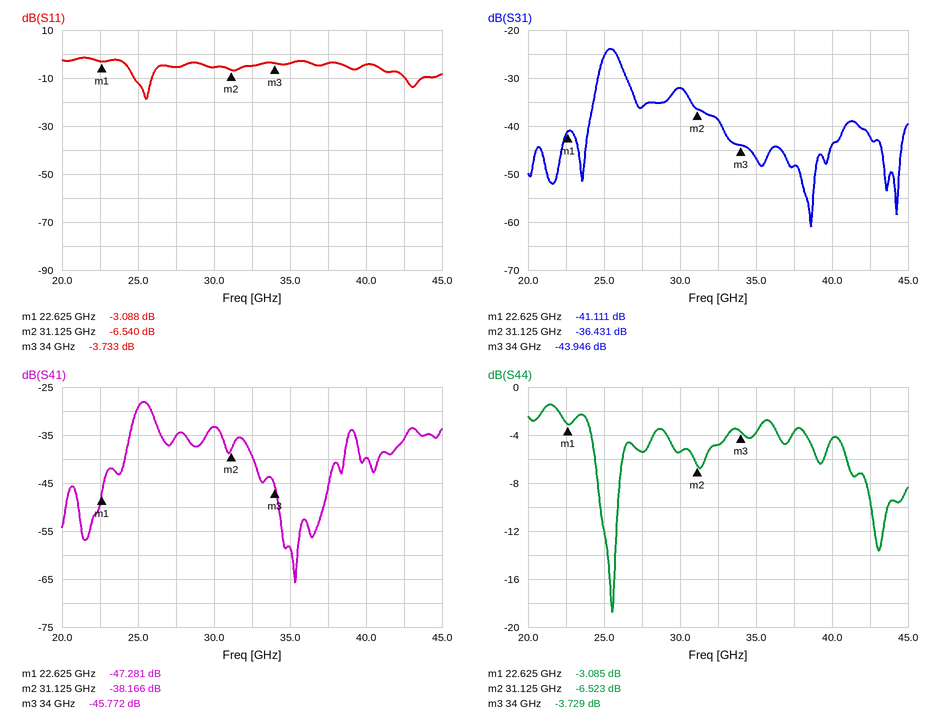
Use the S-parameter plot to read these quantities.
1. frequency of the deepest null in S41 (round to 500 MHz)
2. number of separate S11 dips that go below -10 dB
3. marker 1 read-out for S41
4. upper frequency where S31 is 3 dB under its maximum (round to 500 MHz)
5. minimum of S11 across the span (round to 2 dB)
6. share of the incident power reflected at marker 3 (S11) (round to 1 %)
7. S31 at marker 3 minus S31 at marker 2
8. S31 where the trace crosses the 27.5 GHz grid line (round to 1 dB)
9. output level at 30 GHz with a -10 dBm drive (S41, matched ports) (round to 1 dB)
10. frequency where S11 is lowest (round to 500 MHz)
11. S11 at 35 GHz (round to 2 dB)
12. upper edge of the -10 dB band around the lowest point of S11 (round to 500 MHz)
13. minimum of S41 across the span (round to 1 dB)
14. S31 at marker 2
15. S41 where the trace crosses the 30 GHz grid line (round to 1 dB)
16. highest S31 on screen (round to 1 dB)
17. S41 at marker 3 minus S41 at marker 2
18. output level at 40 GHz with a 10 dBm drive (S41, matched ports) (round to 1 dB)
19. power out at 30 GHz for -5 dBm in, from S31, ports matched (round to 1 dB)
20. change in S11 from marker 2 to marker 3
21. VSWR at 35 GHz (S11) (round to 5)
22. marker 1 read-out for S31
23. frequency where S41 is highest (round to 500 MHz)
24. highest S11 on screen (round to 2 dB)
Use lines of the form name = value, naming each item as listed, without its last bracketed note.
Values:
frequency of the deepest null in S41 = 35.5 GHz
number of separate S11 dips that go below -10 dB = 2
marker 1 read-out for S41 = -47.281 dB
upper frequency where S31 is 3 dB under its maximum = 26.0 GHz
minimum of S11 across the span = -18 dB
share of the incident power reflected at marker 3 (S11) = 42 %
S31 at marker 3 minus S31 at marker 2 = -7.515 dB
S31 where the trace crosses the 27.5 GHz grid line = -36 dB
output level at 30 GHz with a -10 dBm drive (S41, matched ports) = -43 dBm
frequency where S11 is lowest = 25.5 GHz
S11 at 35 GHz = -4 dB
upper edge of the -10 dB band around the lowest point of S11 = 26.0 GHz
minimum of S41 across the span = -66 dB
S31 at marker 2 = -36.431 dB
S41 where the trace crosses the 30 GHz grid line = -33 dB
highest S31 on screen = -24 dB
S41 at marker 3 minus S41 at marker 2 = -7.606 dB
output level at 40 GHz with a 10 dBm drive (S41, matched ports) = -30 dBm
power out at 30 GHz for -5 dBm in, from S31, ports matched = -37 dBm
change in S11 from marker 2 to marker 3 = 2.807 dB
VSWR at 35 GHz (S11) = 5
marker 1 read-out for S31 = -41.111 dB
frequency where S41 is highest = 25.5 GHz
highest S11 on screen = -2 dB
